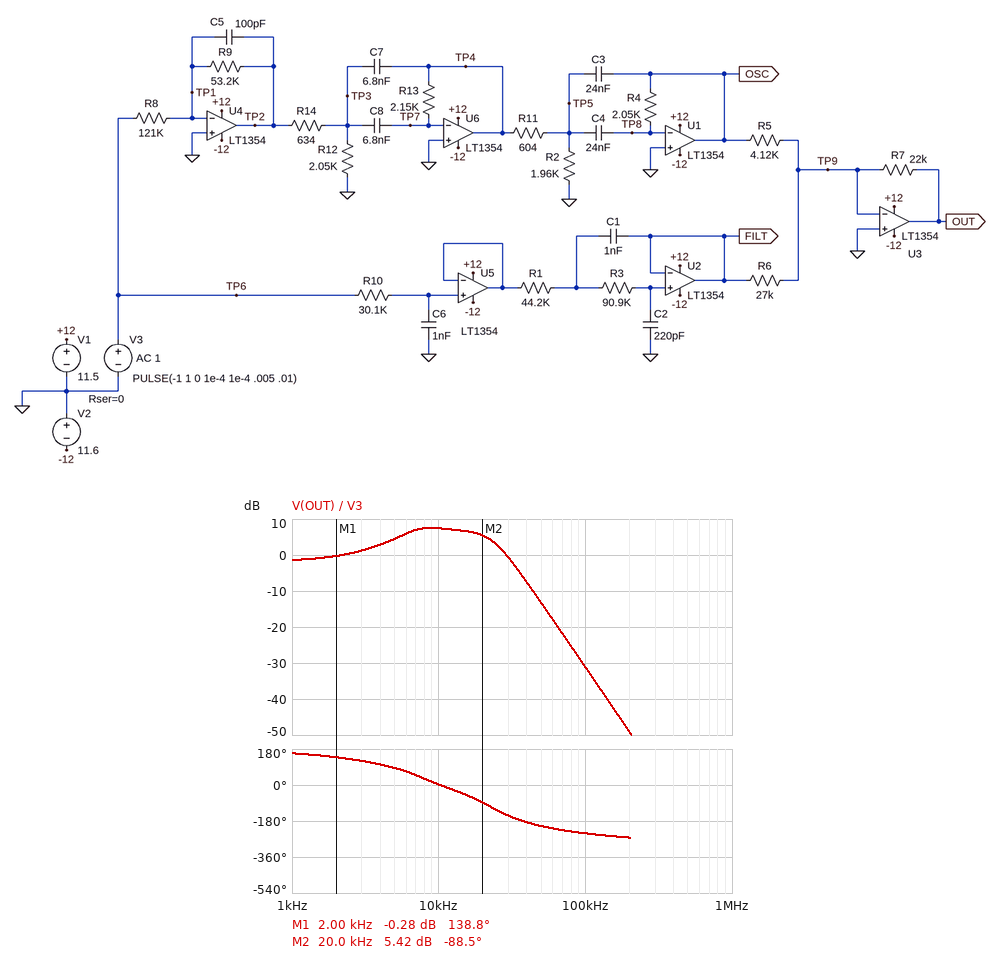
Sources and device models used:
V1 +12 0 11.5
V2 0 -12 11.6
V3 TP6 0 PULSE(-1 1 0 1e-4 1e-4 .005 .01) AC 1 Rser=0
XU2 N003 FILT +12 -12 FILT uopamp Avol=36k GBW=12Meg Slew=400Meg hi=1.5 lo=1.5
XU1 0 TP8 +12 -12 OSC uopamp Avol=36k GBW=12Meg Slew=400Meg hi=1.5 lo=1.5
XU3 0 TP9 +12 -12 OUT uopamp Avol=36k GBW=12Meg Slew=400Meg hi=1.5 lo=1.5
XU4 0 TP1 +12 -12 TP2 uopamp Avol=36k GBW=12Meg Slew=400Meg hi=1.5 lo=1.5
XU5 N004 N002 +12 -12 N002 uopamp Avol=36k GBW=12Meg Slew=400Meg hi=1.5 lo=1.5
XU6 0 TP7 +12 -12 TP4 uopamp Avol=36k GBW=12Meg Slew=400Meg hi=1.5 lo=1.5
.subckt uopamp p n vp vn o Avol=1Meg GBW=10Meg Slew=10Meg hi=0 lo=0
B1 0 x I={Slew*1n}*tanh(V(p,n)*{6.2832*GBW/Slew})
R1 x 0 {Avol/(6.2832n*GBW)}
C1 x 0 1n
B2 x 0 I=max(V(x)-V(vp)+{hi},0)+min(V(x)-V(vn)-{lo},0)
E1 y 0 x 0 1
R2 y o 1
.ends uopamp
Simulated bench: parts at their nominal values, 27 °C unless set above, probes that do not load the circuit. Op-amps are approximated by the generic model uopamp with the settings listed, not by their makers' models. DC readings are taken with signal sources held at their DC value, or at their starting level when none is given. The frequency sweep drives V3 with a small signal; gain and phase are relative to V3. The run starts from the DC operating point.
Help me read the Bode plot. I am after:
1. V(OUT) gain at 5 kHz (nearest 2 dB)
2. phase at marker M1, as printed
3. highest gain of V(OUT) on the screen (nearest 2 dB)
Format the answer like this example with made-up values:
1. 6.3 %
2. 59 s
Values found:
1. 4 dB
2. 138.8 deg
3. 8 dB
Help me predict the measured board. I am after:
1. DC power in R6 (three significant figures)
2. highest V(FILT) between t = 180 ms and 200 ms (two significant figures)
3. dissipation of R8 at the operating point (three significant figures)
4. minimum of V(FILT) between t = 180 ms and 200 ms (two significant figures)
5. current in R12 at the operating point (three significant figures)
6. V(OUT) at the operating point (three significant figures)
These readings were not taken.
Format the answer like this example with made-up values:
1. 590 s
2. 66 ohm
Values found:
1. 37.0 µW
2. 1.1 V
3. 8.26 µW
4. -1.1 V
5. 164 µA
6. 815 mV
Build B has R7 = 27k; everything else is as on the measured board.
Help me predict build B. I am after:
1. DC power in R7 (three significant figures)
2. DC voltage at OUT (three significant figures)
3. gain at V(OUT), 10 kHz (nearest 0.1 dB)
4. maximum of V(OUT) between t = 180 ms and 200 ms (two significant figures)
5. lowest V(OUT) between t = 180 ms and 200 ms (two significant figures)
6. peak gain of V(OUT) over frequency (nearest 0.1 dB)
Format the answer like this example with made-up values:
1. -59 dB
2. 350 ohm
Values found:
1. 37.0 µW
2. 1.00 V
3. 9.2 dB
4. 1.6 V
5. -1.6 V
6. 9.3 dB
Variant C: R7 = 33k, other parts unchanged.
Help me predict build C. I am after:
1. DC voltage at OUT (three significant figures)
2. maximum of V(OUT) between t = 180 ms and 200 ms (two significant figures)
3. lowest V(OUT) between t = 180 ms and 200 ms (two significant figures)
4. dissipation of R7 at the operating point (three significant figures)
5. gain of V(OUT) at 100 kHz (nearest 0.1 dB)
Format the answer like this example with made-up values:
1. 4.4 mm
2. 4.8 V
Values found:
1. 1.22 V
2. 1.9 V
3. -1.9 V
4. 45.2 µW
5. -27.6 dB
